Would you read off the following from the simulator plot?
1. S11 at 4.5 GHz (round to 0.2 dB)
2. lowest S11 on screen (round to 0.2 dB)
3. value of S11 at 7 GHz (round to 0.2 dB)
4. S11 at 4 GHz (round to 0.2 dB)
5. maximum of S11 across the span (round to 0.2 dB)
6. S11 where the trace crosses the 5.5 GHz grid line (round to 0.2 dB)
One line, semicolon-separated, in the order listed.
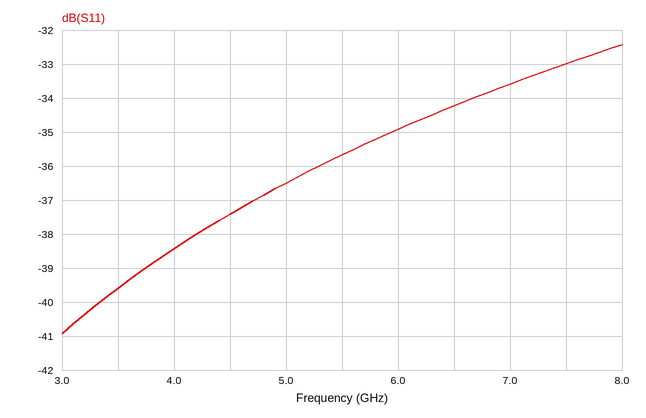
-37.4 dB; -41.0 dB; -33.6 dB; -38.4 dB; -32.4 dB; -35.6 dB
